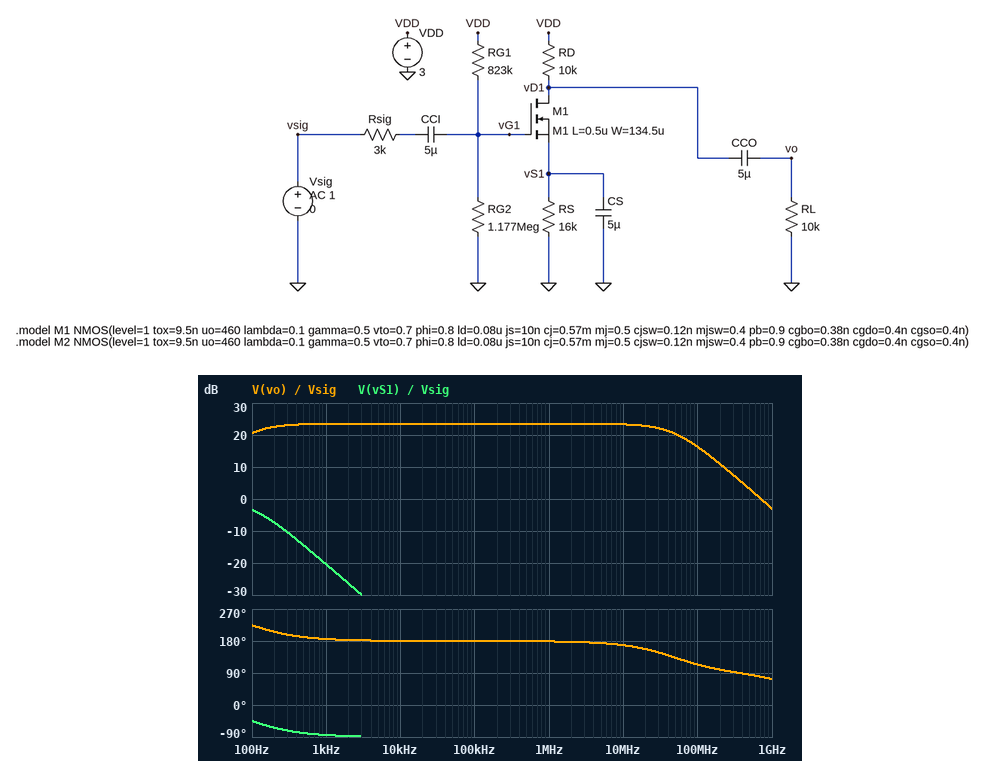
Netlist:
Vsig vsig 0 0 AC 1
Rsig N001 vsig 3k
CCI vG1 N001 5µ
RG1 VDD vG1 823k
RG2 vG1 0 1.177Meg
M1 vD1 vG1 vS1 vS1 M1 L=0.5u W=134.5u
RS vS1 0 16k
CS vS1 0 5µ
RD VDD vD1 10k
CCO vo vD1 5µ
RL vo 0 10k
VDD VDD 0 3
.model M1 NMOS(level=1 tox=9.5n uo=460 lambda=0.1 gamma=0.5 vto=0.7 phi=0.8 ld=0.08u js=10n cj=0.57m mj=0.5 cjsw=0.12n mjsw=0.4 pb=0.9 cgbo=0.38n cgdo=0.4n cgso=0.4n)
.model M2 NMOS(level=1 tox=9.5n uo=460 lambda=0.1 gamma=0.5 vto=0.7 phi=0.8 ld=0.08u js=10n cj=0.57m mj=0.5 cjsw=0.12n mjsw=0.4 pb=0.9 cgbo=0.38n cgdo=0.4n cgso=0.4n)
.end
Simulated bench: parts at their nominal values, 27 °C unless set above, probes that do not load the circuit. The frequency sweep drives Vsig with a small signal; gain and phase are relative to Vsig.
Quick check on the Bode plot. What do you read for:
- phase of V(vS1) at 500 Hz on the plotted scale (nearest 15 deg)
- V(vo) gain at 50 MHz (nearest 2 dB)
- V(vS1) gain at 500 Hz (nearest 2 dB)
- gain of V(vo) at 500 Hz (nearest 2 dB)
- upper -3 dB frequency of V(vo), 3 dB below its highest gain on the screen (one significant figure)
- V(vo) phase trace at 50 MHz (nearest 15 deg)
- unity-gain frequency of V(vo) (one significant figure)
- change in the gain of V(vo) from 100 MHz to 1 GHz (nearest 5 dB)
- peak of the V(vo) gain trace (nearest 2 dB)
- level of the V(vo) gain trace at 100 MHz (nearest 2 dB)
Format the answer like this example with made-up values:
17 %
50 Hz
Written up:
-75 deg
20 dB
-14 dB
24 dB
50 MHz
135 deg
700 MHz
-20 dB
24 dB
16 dB
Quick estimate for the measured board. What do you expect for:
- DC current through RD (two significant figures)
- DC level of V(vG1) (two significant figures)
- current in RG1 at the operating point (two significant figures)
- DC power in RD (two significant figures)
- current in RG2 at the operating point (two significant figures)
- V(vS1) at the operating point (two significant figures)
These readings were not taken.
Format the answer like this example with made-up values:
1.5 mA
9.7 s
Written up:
64 µA
1.8 V
1.5 µA
41 µW
1.5 µA
1.0 V
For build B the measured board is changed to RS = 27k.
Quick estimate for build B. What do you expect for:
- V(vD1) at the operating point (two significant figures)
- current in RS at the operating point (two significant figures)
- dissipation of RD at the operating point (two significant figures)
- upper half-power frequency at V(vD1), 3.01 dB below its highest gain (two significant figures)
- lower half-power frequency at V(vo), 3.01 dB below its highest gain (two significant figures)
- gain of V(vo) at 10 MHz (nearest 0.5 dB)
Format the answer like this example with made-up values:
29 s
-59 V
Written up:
2.6 V
38 µA
15 µW
57 MHz
77 Hz
21.5 dB
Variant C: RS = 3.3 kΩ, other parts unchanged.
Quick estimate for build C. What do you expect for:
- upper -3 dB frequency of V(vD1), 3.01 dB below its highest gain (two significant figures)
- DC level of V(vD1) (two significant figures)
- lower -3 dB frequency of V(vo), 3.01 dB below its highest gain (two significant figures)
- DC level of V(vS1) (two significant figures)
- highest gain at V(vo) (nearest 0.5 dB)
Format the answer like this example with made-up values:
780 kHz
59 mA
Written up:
200 MHz
750 mV
11 Hz
740 mV
-29.5 dB
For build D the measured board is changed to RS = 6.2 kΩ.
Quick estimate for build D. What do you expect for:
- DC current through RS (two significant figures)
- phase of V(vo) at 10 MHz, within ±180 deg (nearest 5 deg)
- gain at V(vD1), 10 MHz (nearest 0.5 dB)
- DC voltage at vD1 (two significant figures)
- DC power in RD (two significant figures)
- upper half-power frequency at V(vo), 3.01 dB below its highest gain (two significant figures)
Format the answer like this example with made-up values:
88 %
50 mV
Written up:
160 µA
165 deg
26.5 dB
1.4 V
260 µW
36 MHz
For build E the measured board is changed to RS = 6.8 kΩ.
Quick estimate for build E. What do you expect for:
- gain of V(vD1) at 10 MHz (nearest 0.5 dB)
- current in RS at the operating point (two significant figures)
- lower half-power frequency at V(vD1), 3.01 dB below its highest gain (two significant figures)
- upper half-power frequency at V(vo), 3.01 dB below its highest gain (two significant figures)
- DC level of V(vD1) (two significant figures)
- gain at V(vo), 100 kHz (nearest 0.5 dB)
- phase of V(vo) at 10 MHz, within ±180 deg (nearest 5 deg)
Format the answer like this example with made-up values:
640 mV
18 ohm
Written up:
26.0 dB
150 µA
140 Hz
37 MHz
1.5 V
26.5 dB
165 deg
